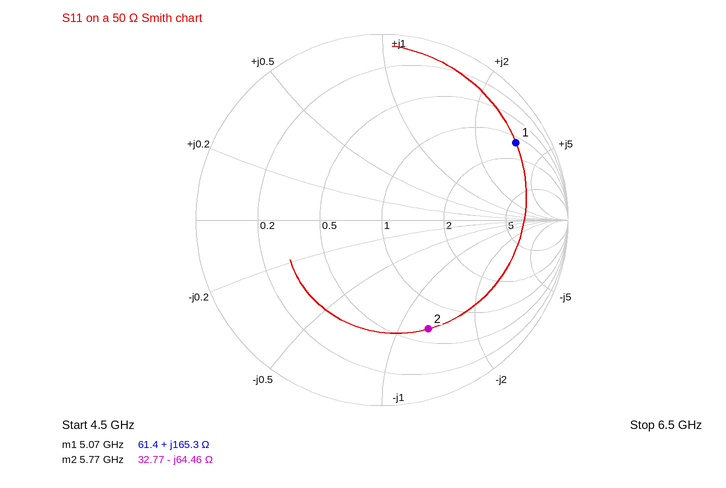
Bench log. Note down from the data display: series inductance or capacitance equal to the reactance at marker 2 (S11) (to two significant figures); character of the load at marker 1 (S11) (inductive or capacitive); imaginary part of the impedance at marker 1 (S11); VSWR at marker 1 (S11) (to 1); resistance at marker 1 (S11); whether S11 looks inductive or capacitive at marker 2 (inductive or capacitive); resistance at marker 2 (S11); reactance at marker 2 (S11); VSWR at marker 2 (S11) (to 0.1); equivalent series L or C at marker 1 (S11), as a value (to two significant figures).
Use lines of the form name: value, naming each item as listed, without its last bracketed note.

series inductance or capacitance equal to the reactance at marker 2 (S11): 430 fF
character of the load at marker 1 (S11): inductive
imaginary part of the impedance at marker 1: +165.3 Ω
VSWR at marker 1 (S11): 11
resistance at marker 1: 61.4 Ω
whether S11 looks inductive or capacitive at marker 2: capacitive
resistance at marker 2: 32.77 Ω
reactance at marker 2: -64.46 Ω
VSWR at marker 2 (S11): 4.5
equivalent series L or C at marker 1 (S11), as a value: 5.2 nH
